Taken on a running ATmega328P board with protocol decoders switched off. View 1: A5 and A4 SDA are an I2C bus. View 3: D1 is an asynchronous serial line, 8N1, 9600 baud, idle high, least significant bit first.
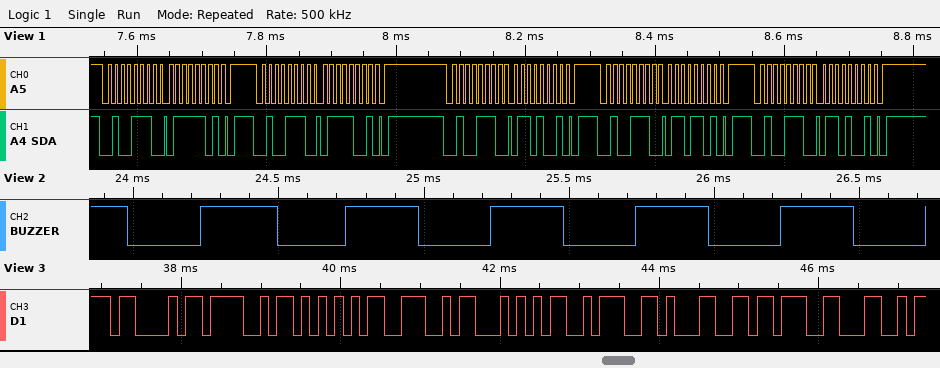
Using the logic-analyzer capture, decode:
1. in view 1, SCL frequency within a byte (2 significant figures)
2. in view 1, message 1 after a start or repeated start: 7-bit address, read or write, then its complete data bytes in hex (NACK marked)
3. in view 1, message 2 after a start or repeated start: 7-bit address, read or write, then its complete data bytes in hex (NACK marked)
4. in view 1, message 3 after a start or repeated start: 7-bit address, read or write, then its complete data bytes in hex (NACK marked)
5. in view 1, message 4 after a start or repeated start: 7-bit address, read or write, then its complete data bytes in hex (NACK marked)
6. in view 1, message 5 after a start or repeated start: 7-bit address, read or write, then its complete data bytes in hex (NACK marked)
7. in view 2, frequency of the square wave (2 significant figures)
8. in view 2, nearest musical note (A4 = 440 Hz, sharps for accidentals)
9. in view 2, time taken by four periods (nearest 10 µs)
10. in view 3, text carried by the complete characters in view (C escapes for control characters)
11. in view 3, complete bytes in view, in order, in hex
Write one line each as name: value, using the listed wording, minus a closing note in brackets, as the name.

in view 1, SCL frequency within a byte: 100 kHz
in view 1, message 1 after a start or repeated start: 7-bit address, read or write, then its complete data bytes in hex: 0x27 write: 7D
in view 1, message 2 after a start or repeated start: 7-bit address, read or write, then its complete data bytes in hex: 0x27 write: 79
in view 1, message 3 after a start or repeated start: 7-bit address, read or write, then its complete data bytes in hex: 0x27 write: 69
in view 1, message 4 after a start or repeated start: 7-bit address, read or write, then its complete data bytes in hex: 0x27 write: 6D
in view 1, message 5 after a start or repeated start: 7-bit address, read or write, then its complete data bytes in hex: 0x27 write: 69
in view 2, frequency of the square wave: 2.0 kHz
in view 2, nearest musical note: B6
in view 2, time taken by four periods: 2000 µs
in view 3, text carried by the complete characters in view: "COUNT:1;L"
in view 3, complete bytes in view, in order, in hex: 43 4F 55 4E 54 3A 31 3B 4C
